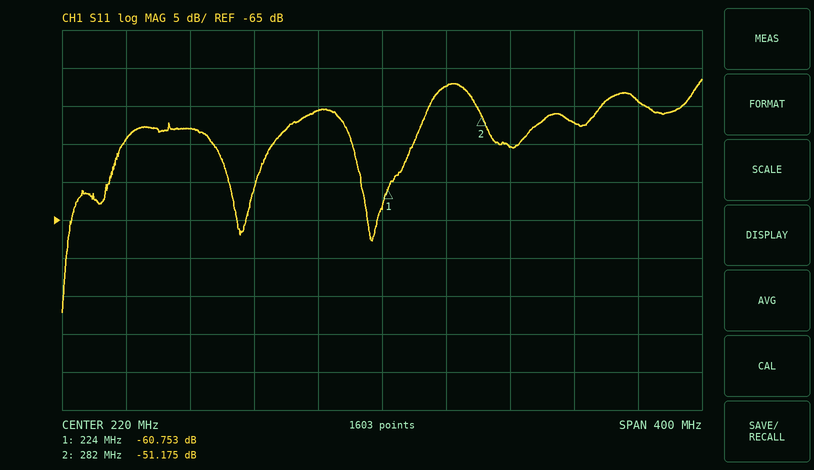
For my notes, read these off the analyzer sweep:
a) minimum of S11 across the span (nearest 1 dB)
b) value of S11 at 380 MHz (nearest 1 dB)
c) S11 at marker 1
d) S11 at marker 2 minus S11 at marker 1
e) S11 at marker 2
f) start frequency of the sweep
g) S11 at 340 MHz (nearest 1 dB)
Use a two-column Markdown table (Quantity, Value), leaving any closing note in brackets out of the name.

| Quantity | Value |
|---|---|
| minimum of S11 across the span | -77 dB |
| value of S11 at 380 MHz | -49 dB |
| S11 at marker 1 | -60.753 dB |
| S11 at marker 2 minus S11 at marker 1 | 9.578 dB |
| S11 at marker 2 | -51.175 dB |
| start frequency of the sweep | 20 MHz |
| S11 at 340 MHz | -52 dB |
